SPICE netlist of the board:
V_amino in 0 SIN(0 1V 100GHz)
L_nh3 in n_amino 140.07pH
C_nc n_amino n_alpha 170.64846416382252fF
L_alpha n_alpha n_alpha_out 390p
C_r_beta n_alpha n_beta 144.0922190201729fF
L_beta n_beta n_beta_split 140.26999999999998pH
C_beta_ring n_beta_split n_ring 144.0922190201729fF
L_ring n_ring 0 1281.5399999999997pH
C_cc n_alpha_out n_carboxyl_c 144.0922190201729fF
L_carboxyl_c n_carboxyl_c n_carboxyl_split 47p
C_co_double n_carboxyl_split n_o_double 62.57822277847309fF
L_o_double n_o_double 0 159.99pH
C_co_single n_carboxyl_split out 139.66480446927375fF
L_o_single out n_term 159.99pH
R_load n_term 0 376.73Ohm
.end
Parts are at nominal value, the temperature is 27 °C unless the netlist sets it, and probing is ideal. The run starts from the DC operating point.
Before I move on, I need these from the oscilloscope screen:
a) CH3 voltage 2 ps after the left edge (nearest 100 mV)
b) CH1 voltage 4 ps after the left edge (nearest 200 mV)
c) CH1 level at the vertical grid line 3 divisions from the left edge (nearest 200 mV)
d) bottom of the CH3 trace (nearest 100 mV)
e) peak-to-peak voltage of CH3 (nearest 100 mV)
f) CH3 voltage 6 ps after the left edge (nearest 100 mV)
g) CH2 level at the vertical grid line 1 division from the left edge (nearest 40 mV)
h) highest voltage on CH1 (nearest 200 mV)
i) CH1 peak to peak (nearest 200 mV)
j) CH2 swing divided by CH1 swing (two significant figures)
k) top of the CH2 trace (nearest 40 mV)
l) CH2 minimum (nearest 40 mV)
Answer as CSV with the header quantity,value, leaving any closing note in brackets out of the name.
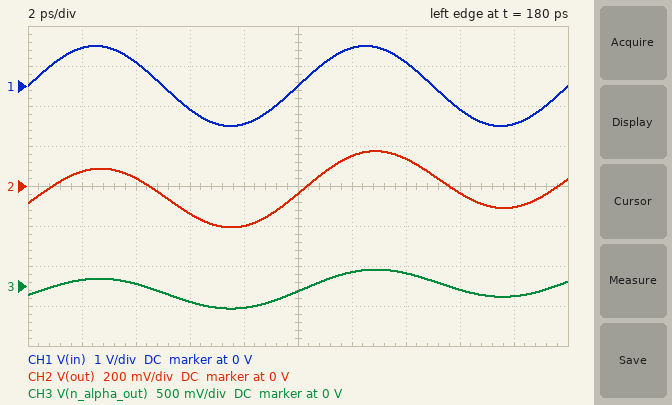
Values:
quantity,value
CH3 voltage 2 ps after the left edge,100 mV
CH1 voltage 4 ps after the left edge,600 mV
CH1 level at the vertical grid line 3 divisions from the left edge,-600 mV
bottom of the CH3 trace,-300 mV
peak-to-peak voltage of CH3,500 mV
CH3 voltage 6 ps after the left edge,-200 mV
CH2 level at the vertical grid line 1 division from the left edge,80 mV
highest voltage on CH1,1.0 V
CH1 peak to peak,2.0 V
CH2 swing divided by CH1 swing,0.19
top of the CH2 trace,160 mV
CH2 minimum,-200 mV
